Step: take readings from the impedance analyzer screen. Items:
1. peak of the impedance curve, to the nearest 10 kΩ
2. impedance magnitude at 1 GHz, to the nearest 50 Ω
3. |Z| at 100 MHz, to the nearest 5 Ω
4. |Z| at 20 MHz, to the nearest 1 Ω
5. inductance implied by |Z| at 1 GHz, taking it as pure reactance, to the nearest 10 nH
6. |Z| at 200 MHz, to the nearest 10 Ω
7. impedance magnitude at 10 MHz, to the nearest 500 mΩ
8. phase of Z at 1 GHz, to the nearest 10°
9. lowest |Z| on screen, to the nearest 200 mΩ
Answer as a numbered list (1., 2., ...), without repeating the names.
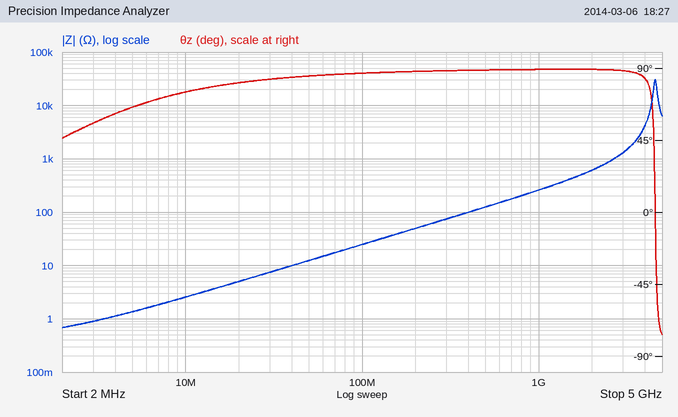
1. 30 kΩ
2. 250 Ω
3. 25 Ω
4. 5 Ω
5. 40 nH
6. 50 Ω
7. 2.5 Ω
8. 90°
9. 600 mΩ
